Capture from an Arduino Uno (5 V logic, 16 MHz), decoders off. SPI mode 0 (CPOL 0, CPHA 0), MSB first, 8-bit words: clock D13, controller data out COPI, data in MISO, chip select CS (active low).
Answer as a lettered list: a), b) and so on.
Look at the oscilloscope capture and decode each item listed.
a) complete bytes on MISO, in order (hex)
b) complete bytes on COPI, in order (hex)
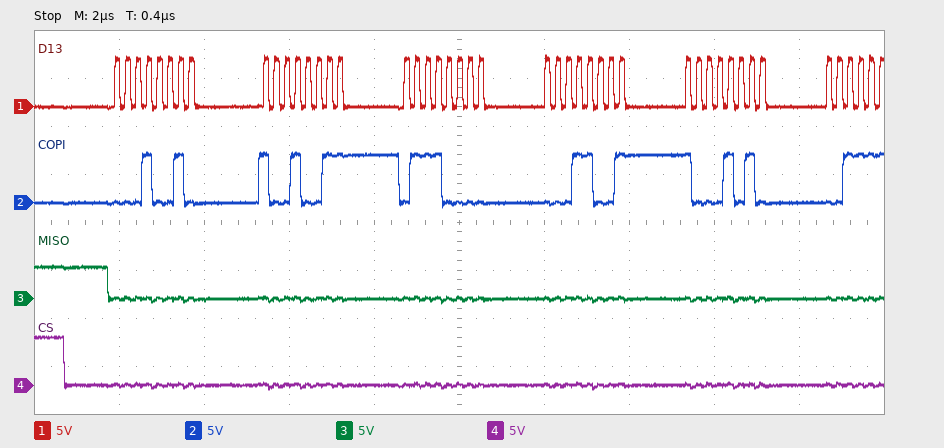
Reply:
a) 00 00 00 00 00
b) 12 93 70 19 8A
